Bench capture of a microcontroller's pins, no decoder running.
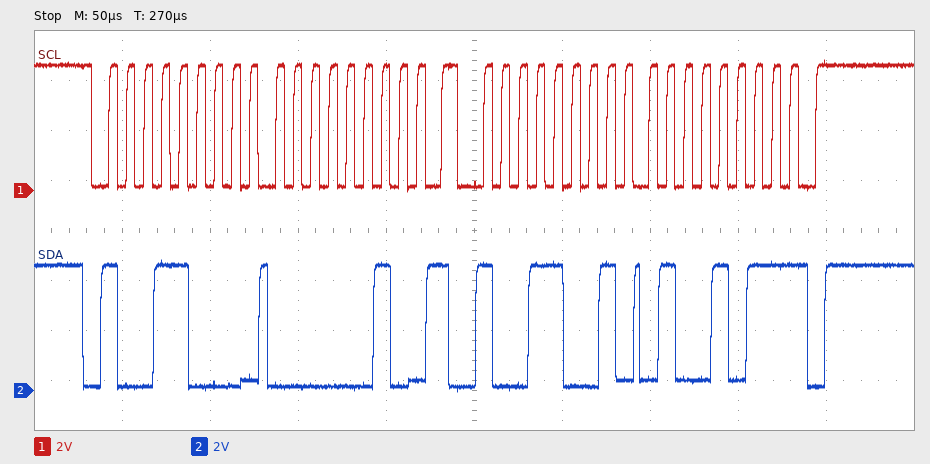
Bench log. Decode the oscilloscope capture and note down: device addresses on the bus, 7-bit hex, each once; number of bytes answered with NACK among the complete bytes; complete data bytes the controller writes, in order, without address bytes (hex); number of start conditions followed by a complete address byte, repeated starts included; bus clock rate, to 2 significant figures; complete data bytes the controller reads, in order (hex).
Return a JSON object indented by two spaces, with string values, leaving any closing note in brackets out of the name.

{
  "device addresses on the bus, 7-bit hex, each once": "0x4C",
  "number of bytes answered with NACK among the complete bytes": "1",
  "complete data bytes the controller writes, in order, without address bytes": "02",
  "number of start conditions followed by a complete address byte, repeated starts included": "2",
  "bus clock rate, to 2 significant figures": "100 kHz",
  "complete data bytes the controller reads, in order": "4B"
}
